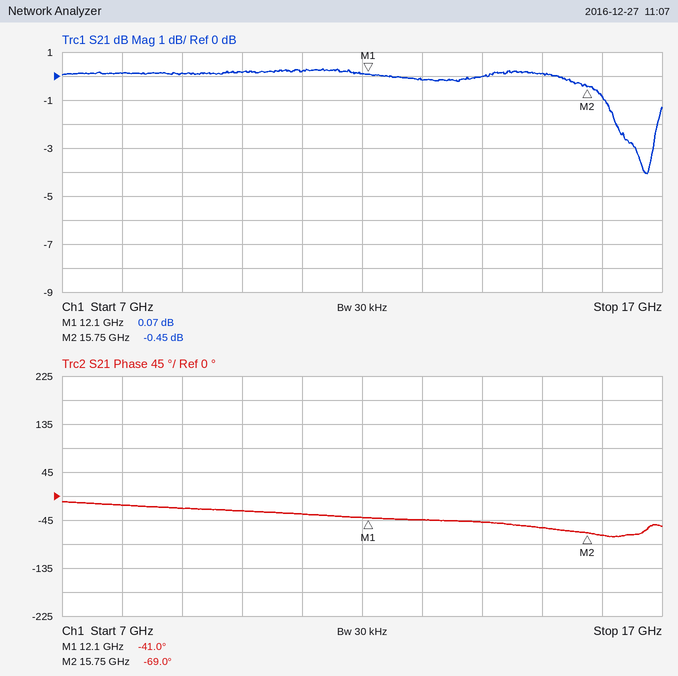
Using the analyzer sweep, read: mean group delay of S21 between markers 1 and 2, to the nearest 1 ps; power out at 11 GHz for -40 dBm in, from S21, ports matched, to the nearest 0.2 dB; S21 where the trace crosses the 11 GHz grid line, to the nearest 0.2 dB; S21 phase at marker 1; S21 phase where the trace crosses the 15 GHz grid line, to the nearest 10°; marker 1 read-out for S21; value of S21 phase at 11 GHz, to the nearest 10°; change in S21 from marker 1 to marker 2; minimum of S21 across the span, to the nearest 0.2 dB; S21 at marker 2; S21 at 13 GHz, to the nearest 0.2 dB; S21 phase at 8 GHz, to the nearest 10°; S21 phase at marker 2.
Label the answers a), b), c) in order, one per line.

a) 21 ps
b) -39.8 dBm
c) 0.2 dB
d) -41.0°
e) -60°
f) 0.07 dB
g) -30°
h) -0.52 dB
i) -4.0 dB
j) -0.45 dB
k) -0.2 dB
l) -20°
m) -69.0°
